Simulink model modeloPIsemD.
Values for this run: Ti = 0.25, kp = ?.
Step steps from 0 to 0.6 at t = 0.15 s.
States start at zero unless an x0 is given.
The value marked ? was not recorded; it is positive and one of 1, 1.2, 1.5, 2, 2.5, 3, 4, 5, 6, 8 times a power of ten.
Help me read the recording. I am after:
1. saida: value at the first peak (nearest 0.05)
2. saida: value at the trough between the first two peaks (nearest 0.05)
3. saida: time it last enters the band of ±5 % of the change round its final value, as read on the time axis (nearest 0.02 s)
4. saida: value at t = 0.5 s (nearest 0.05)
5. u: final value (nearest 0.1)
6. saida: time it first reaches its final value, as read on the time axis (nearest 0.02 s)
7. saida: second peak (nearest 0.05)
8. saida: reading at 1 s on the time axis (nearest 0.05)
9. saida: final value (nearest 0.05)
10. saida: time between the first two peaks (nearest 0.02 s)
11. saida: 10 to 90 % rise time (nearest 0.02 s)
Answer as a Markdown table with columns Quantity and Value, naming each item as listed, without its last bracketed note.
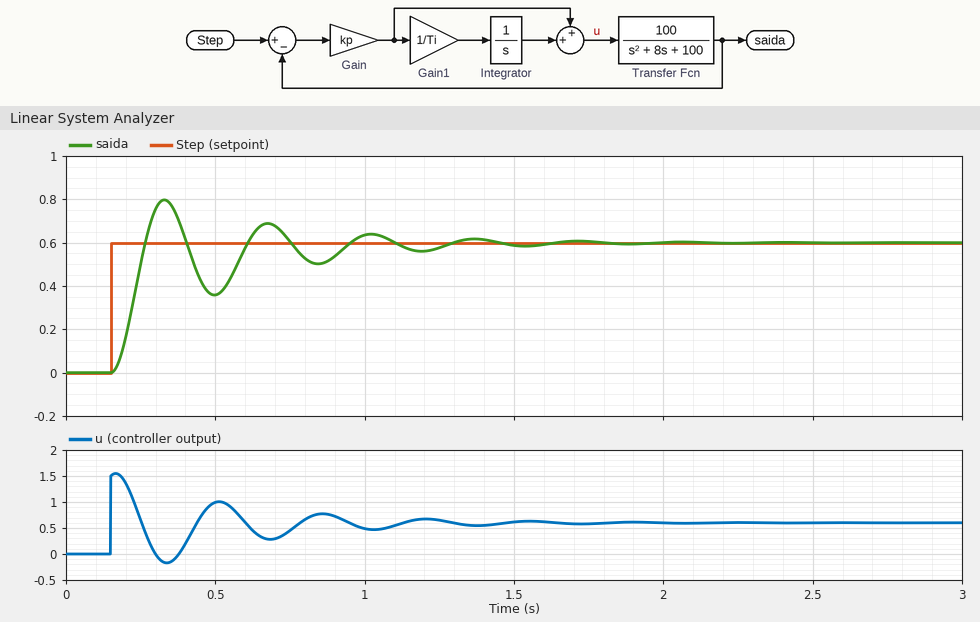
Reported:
| Quantity | Value |
|---|---|
| saida: value at the first peak | 0.80 |
| saida: value at the trough between the first two peaks | 0.35 |
| saida: time it last enters the band of ±5 % of the change round its final value, as read on the time axis | 1.24 s |
| saida: value at t = 0.5 s | 0.35 |
| u: final value | 0.6 |
| saida: time it first reaches its final value, as read on the time axis | 0.26 s |
| saida: second peak | 0.70 |
| saida: reading at 1 s on the time axis | 0.65 |
| saida: final value | 0.60 |
| saida: time between the first two peaks | 0.34 s |
| saida: 10 to 90 % rise time | 0.08 s |
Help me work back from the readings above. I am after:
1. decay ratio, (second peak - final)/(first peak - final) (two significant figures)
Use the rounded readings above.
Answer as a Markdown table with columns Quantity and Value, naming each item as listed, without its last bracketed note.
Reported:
| Quantity | Value |
|---|---|
| decay ratio, (second peak - final)/(first peak - final) | 0.50 |
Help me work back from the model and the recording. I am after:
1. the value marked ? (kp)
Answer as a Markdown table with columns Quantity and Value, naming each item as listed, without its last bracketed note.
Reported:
| Quantity | Value |
|---|---|
| the value marked ? | 2.5 |
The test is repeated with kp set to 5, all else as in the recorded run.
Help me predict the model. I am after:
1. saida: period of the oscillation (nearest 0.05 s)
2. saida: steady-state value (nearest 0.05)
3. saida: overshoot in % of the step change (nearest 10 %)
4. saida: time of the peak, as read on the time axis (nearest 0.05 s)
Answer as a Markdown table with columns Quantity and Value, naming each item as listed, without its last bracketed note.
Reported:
| Quantity | Value |
|---|---|
| saida: period of the oscillation | 0.25 s |
| saida: steady-state value | 0.60 |
| saida: overshoot in % of the step change | 50 % |
| saida: time of the peak, as read on the time axis | 0.30 s |
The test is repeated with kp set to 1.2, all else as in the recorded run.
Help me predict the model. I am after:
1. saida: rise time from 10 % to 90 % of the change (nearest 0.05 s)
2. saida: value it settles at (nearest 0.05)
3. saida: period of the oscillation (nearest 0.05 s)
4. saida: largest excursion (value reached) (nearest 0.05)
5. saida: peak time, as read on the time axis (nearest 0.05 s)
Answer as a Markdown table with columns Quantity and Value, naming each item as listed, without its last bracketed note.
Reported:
| Quantity | Value |
|---|---|
| saida: rise time from 10 % to 90 % of the change | 0.15 s |
| saida: value it settles at | 0.60 |
| saida: period of the oscillation | 0.45 s |
| saida: largest excursion (value reached) | 0.65 |
| saida: peak time, as read on the time axis | 0.40 s |
